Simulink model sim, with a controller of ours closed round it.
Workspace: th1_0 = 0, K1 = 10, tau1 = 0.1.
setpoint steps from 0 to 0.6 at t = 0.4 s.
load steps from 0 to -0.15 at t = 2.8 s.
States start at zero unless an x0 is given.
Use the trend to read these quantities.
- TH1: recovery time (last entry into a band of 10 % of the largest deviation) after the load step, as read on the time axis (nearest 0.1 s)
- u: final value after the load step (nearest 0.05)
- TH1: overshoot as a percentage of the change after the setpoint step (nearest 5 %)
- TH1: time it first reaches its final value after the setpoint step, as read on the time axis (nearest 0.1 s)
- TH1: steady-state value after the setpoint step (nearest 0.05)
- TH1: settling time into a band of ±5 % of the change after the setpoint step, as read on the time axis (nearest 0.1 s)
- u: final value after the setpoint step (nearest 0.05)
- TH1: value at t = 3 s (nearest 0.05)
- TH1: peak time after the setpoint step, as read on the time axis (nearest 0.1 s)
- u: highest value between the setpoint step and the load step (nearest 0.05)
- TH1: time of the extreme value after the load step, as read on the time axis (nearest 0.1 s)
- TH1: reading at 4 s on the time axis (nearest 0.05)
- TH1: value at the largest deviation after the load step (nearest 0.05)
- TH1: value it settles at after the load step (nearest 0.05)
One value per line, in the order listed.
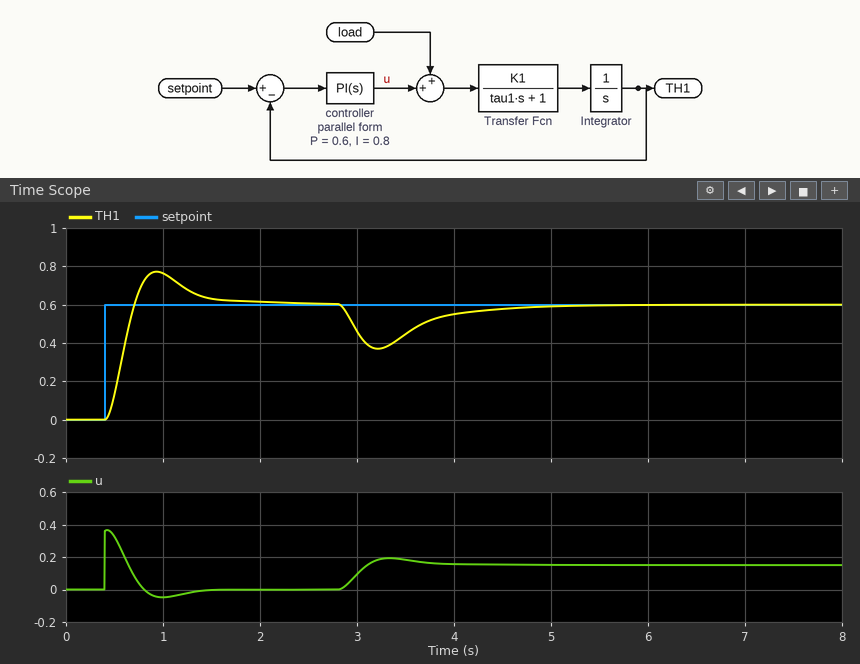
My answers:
4.5 s
0.15
30 %
0.7 s
0.60
1.5 s
0.00
0.45
0.9 s
0.35
3.2 s
0.55
0.35
0.60
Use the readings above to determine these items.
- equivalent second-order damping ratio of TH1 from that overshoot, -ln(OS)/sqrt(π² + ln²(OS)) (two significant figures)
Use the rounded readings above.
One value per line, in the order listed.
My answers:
0.36
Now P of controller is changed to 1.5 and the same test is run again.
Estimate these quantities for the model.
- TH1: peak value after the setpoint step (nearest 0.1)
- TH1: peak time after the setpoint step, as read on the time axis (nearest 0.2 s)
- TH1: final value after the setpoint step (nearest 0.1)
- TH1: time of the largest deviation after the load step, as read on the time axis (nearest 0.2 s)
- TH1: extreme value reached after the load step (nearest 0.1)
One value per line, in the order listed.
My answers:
0.8
0.6 s
0.6
3.0 s
0.5
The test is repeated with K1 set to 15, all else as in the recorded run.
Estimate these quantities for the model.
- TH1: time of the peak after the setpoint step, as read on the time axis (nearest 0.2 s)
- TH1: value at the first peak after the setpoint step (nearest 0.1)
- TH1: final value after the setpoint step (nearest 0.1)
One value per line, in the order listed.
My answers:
0.8 s
0.8
0.6
